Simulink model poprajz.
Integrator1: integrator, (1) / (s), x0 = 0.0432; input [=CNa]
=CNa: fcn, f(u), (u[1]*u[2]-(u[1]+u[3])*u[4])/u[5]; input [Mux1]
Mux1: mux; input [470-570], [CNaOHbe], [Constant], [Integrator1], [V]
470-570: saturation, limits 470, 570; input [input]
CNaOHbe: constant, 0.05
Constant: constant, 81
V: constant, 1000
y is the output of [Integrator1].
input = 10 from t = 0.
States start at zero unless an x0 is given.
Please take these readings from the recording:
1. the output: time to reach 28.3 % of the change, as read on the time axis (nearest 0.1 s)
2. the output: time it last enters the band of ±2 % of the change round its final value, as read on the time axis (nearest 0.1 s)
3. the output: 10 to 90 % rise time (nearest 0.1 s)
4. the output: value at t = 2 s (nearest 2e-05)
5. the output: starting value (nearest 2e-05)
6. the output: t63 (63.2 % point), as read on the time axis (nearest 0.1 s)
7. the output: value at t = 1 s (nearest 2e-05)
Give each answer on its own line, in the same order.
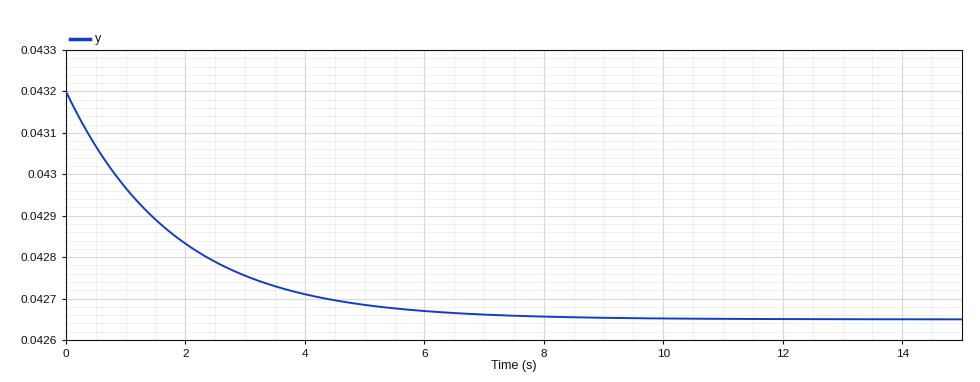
0.6 s
7.1 s
4.0 s
0.04284
0.04320
1.8 s
0.04296
